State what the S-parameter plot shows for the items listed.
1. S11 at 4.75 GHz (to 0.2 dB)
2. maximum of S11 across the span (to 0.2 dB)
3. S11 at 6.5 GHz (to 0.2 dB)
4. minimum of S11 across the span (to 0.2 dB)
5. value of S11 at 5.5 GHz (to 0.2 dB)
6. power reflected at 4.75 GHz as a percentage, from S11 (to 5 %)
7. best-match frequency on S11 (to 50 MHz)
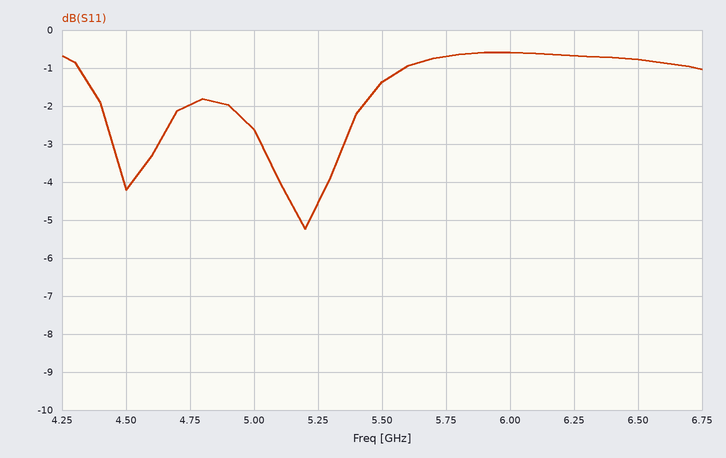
-2.0 dB
-0.6 dB
-0.8 dB
-5.2 dB
-1.4 dB
65 %
5.20 GHz
